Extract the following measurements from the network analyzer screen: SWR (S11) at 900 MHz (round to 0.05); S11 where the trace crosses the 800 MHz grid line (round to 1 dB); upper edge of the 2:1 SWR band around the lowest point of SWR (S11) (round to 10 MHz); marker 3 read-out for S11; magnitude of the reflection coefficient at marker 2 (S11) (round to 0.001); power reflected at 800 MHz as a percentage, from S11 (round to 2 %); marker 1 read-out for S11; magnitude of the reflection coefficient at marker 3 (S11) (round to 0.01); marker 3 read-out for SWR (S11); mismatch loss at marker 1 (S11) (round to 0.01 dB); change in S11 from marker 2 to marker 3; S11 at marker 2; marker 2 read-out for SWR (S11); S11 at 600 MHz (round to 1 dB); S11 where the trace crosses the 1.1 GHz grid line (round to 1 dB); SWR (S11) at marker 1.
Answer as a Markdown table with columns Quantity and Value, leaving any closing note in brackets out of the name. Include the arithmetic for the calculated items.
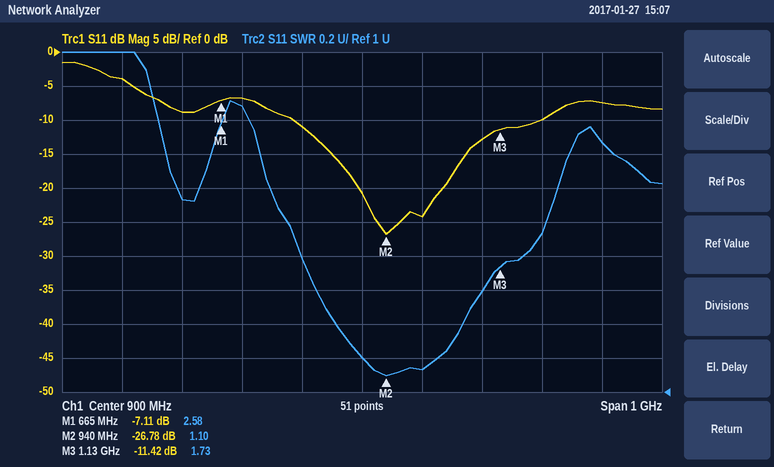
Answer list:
| Quantity | Value |
|---|---|
| SWR (S11) at 900 MHz | 1.20 |
| S11 where the trace crosses the 800 MHz grid line | -11 dB |
| upper edge of the 2:1 SWR band around the lowest point of SWR (S11) | 1.21 GHz |
| marker 3 read-out for S11 | -11.42 dB |
| magnitude of the reflection coefficient at marker 2 (S11) | 10^(-26.78/20) ≈ 0.046 |
| power reflected at 800 MHz as a percentage, from S11 | 10^(-11/10) ≈ 8 % |
| marker 1 read-out for S11 | -7.11 dB |
| magnitude of the reflection coefficient at marker 3 (S11) | 10^(-11.42/20) ≈ 0.27 |
| marker 3 read-out for SWR | 1.73 |
| mismatch loss at marker 1 (S11) | −10 log10(1 − 10^(-7.11/10)) ≈ 0.94 dB |
| change in S11 from marker 2 to marker 3 | -11.42 − (-26.78) = 15.36 dB |
| S11 at marker 2 | -26.78 dB |
| marker 2 read-out for SWR | 1.10 |
| S11 at 600 MHz | -9 dB |
| S11 where the trace crosses the 1.1 GHz grid line | -13 dB |
| SWR (S11) at marker 1 | 2.58 |
